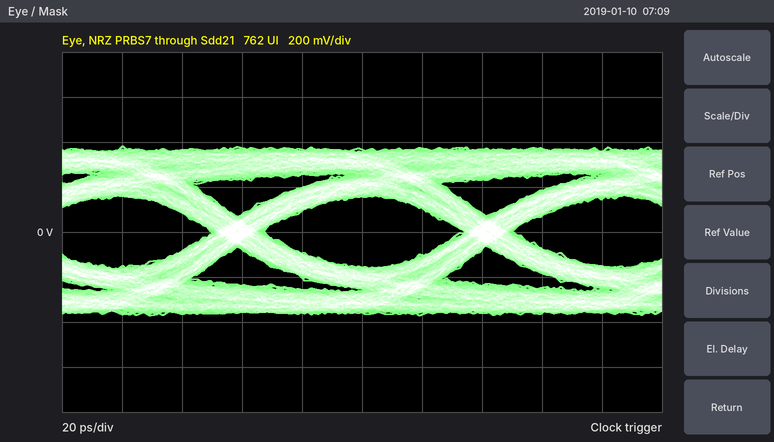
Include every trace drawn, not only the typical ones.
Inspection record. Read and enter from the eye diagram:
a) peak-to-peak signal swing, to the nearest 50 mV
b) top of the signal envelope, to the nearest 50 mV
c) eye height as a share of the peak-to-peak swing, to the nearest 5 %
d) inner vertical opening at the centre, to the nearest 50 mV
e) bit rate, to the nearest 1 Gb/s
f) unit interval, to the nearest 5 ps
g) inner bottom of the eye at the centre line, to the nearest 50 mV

750 mV
400 mV
40 %
300 mV
12 Gb/s
85 ps
-150 mV
